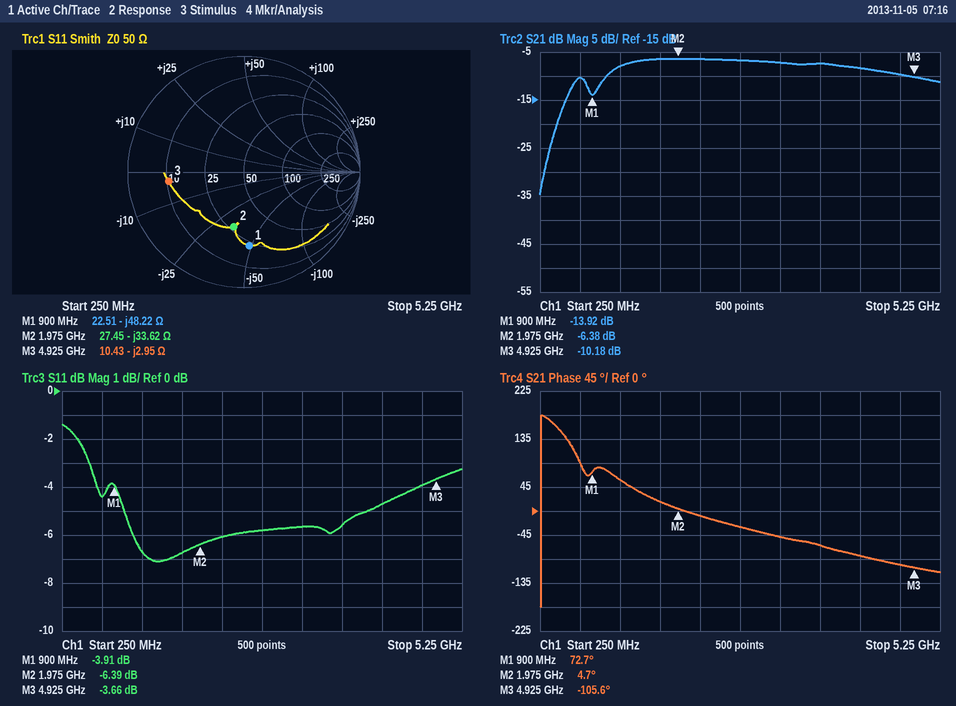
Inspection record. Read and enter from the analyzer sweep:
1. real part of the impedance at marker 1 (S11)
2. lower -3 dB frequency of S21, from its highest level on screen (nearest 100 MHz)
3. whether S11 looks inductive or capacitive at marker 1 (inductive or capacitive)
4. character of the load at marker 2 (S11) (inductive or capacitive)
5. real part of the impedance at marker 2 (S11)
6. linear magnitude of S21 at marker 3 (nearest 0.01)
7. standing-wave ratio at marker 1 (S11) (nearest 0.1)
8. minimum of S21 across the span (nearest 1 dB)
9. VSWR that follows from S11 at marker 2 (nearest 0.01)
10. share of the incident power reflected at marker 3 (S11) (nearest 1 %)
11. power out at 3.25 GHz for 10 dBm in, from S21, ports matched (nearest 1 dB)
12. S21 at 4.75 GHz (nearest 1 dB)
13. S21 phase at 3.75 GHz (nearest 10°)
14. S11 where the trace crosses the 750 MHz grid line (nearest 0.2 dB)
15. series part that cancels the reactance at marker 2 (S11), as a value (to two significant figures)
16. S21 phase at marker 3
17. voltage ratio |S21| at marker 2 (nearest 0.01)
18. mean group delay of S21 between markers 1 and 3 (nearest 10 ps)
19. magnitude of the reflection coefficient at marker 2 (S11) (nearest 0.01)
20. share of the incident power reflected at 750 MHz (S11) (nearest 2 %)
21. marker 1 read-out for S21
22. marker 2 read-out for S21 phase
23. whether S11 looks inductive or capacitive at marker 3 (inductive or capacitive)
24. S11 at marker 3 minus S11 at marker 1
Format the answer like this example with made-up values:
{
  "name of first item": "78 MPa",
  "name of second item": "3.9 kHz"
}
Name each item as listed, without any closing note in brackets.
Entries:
{
  "real part of the impedance at marker 1": "22.51 Ω",
  "lower -3 dB frequency of S21, from its highest level on screen": "1.1 GHz",
  "whether S11 looks inductive or capacitive at marker 1": "capacitive",
  "character of the load at marker 2 (S11)": "capacitive",
  "real part of the impedance at marker 2": "27.45 Ω",
  "linear magnitude of S21 at marker 3": "0.31",
  "standing-wave ratio at marker 1 (S11)": "4.5",
  "minimum of S21 across the span": "-35 dB",
  "VSWR that follows from S11 at marker 2": "2.84",
  "share of the incident power reflected at marker 3 (S11)": "43 %",
  "power out at 3.25 GHz for 10 dBm in, from S21, ports matched": "3 dBm",
  "S21 at 4.75 GHz": "-10 dB",
  "S21 phase at 3.75 GHz": "-60°",
  "S11 where the trace crosses the 750 MHz grid line": "-4.4 dB",
  "series part that cancels the reactance at marker 2 (S11), as a value": "2.7 nH",
  "S21 phase at marker 3": "-105.6°",
  "voltage ratio |S21| at marker 2": "0.48",
  "mean group delay of S21 between markers 1 and 3": "120 ps",
  "magnitude of the reflection coefficient at marker 2 (S11)": "0.48",
  "share of the incident power reflected at 750 MHz (S11)": "36 %",
  "marker 1 read-out for S21": "-13.92 dB",
  "marker 2 read-out for S21 phase": "4.7°",
  "whether S11 looks inductive or capacitive at marker 3": "capacitive",
  "S11 at marker 3 minus S11 at marker 1": "0.25 dB"
}
